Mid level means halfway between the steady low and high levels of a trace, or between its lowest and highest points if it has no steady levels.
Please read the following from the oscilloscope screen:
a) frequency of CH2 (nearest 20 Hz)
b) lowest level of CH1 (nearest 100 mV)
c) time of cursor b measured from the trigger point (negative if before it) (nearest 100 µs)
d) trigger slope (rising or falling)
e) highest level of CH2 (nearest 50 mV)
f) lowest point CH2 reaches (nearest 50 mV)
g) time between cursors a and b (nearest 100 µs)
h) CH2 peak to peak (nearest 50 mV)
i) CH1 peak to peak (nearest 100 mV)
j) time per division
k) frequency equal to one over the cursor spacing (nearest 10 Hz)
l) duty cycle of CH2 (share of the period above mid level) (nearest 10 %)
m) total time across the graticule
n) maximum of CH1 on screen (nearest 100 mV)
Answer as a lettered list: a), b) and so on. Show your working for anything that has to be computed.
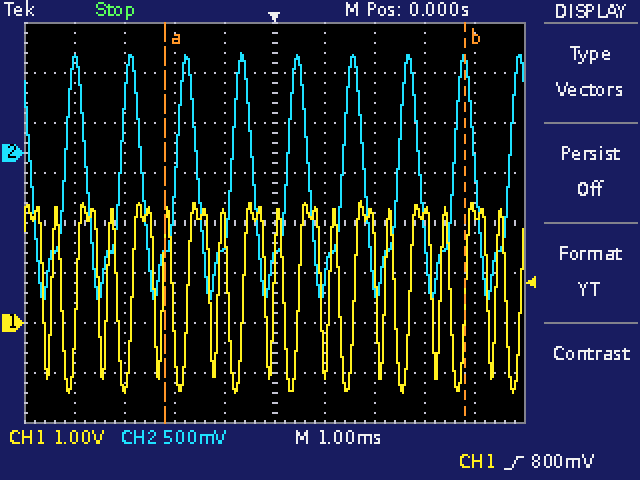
a) 900 Hz
b) -1.4 V
c) +3.8 ms
d) rising
e) 1.00 V
f) -1.45 V
g) 6.0 ms
h) 1.00 V − (-1.45 V) = 2.45 V
i) 2.4 V − (-1.4 V) = 3.8 V
j) 1 ms
k) 1 / 6.0 ms ≈ 170 Hz
l) 40 %
m) 10 ms
n) 2.4 V
